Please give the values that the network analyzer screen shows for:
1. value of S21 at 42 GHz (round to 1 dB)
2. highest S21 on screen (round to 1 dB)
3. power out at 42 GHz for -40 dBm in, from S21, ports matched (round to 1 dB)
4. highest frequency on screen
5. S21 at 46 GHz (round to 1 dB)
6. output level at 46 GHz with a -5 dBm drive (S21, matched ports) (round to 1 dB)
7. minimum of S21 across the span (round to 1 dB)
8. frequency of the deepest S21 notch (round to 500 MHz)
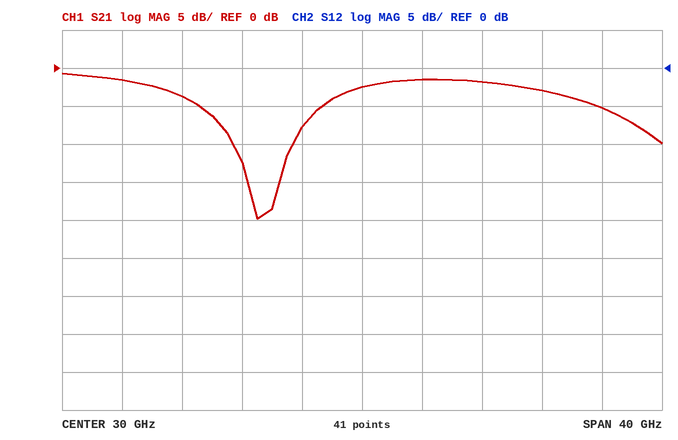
-3 dB
-1 dB
-43 dBm
50 GHz
-5 dB
-10 dBm
-20 dB
23.0 GHz
